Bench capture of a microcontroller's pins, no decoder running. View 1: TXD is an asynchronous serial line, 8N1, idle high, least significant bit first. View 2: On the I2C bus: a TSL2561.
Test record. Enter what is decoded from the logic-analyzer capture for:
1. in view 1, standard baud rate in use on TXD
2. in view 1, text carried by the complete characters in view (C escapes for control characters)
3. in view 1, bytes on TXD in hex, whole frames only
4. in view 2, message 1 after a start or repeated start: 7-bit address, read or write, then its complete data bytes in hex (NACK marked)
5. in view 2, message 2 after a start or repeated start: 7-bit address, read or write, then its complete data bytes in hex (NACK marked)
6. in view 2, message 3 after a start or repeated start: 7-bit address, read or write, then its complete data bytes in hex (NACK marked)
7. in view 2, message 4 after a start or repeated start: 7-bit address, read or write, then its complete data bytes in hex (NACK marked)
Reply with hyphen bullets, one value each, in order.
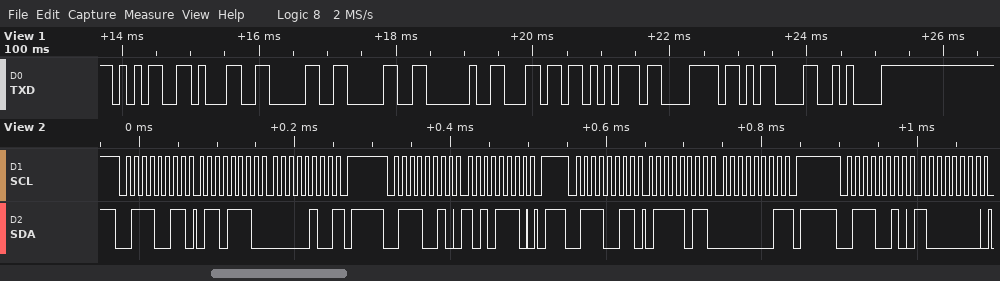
- 9600 baud
- "5100 lux\r\n"
- 35 31 30 30 20 6C 75 78 0D 0A
- 0x39 read: 6E 04 NACK
- 0x39 write: AE
- 0x39 read: 7B 01 NACK
- 0x39 write: 80
